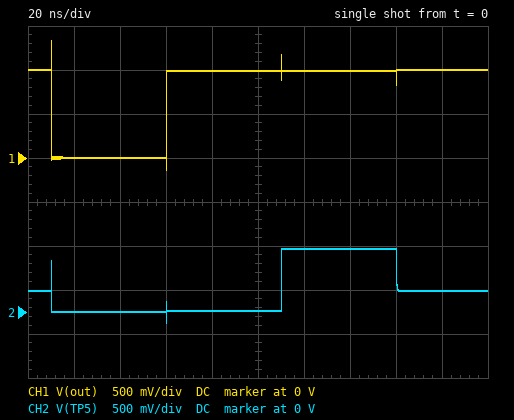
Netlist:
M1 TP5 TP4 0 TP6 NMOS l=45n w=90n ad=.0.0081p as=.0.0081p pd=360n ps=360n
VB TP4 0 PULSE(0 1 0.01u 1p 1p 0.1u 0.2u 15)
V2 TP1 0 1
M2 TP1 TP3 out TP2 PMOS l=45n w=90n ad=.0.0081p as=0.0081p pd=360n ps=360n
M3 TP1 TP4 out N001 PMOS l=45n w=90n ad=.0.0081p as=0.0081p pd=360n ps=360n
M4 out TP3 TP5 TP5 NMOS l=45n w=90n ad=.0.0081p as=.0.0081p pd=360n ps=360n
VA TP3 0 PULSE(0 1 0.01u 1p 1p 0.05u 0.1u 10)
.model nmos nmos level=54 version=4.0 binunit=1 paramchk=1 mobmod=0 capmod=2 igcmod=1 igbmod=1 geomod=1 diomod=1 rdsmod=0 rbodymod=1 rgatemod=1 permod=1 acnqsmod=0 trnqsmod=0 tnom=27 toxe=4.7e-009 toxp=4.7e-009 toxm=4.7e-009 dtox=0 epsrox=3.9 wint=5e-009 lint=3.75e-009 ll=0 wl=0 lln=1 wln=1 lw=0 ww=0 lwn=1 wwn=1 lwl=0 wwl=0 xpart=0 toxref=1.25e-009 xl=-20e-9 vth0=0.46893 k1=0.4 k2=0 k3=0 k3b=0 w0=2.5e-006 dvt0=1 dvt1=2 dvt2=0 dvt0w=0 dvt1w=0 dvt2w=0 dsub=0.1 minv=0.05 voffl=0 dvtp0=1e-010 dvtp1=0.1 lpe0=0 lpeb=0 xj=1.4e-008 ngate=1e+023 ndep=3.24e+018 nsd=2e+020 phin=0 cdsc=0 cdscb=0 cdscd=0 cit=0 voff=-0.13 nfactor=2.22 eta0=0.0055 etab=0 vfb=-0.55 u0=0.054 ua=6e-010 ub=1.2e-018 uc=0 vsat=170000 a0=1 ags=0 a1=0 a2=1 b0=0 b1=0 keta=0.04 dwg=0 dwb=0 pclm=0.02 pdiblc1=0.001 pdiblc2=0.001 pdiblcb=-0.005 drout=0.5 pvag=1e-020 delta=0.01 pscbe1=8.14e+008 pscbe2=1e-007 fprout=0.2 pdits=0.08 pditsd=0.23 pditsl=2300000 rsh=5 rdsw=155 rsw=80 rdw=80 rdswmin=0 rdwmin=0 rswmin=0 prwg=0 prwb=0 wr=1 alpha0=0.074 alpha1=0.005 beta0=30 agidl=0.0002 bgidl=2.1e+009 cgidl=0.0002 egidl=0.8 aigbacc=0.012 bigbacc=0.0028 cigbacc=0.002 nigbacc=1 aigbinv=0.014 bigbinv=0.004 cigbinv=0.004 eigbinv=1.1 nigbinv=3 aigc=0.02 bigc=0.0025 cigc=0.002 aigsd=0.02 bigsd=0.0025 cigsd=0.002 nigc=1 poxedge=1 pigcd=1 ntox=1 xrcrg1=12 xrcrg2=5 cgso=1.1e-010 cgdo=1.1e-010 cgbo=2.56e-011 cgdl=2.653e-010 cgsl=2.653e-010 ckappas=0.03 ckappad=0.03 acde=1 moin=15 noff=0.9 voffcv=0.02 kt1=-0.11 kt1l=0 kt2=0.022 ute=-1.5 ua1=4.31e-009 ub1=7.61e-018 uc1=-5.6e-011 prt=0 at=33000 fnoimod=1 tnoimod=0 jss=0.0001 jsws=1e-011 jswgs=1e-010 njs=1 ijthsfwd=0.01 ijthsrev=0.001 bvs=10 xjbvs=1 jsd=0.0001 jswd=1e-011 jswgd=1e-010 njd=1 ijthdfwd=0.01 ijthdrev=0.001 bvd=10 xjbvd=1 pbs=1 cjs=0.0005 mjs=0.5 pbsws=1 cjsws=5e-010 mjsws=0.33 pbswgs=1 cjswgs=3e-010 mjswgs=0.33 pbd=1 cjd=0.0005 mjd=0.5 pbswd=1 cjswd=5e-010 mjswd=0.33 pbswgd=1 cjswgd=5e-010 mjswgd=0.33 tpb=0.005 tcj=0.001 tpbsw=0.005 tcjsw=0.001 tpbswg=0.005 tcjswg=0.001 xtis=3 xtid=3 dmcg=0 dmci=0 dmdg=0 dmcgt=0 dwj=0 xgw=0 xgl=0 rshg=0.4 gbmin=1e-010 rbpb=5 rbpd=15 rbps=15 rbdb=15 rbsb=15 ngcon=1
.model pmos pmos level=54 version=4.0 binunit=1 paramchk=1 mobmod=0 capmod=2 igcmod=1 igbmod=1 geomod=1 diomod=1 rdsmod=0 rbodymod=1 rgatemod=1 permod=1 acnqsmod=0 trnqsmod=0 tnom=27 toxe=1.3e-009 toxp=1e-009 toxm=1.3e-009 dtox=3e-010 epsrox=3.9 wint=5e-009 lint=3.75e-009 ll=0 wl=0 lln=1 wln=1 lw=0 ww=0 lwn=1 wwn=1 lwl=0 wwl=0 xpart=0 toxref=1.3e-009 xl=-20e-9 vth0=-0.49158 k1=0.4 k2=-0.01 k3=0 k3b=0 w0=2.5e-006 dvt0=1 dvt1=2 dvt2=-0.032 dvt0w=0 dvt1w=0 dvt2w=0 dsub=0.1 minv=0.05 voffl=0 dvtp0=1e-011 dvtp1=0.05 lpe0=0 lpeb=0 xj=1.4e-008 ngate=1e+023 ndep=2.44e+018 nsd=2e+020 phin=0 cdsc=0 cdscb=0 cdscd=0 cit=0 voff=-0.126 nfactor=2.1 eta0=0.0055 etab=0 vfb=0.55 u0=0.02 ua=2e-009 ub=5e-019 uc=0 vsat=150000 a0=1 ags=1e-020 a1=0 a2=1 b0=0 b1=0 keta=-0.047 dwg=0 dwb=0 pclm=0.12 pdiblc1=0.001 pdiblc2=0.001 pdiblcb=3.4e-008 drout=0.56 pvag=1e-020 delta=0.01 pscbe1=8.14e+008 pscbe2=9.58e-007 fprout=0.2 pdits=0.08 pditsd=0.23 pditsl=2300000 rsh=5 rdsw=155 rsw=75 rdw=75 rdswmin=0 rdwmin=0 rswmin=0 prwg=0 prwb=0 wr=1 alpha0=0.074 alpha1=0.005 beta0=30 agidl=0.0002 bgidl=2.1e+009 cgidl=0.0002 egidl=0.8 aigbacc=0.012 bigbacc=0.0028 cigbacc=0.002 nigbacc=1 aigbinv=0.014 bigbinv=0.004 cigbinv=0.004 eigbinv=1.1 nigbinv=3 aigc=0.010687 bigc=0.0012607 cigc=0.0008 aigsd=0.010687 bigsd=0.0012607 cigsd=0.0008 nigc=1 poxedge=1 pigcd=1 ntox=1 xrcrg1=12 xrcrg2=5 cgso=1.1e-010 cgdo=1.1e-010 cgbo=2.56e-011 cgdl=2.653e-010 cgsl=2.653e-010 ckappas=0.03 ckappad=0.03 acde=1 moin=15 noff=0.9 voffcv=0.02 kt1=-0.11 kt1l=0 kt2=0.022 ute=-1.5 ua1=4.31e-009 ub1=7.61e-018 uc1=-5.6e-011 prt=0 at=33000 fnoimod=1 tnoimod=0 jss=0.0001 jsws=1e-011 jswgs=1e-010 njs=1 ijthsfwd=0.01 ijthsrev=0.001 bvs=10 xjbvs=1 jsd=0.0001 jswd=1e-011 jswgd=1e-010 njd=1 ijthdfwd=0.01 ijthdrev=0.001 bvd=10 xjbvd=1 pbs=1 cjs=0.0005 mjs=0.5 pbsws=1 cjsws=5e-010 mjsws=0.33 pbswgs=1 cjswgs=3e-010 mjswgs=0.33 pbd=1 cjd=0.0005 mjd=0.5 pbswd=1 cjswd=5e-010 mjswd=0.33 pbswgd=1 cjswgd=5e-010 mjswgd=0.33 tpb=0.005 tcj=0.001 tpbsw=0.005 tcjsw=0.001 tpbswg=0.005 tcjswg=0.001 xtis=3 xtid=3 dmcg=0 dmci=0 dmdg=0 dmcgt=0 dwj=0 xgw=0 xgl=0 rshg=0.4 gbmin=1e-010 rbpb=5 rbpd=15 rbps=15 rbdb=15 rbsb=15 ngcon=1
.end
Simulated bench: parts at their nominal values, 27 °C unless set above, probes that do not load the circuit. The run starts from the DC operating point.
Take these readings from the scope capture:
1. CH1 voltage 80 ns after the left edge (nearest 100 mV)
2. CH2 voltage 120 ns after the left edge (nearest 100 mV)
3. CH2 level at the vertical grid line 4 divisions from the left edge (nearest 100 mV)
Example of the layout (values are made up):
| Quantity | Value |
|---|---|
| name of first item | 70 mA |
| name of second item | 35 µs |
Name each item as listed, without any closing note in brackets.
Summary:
| Quantity | Value |
|---|---|
| CH1 voltage 80 ns after the left edge | 1.0 V |
| CH2 voltage 120 ns after the left edge | 700 mV |
| CH2 level at the vertical grid line 4 divisions from the left edge | 0 V |
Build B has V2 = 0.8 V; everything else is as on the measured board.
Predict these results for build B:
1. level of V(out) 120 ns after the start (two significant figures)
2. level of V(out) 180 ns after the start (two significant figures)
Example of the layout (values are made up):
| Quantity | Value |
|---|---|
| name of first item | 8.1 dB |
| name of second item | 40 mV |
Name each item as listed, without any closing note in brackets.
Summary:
| Quantity | Value |
|---|---|
| level of V(out) 120 ns after the start | 790 mV |
| level of V(out) 180 ns after the start | 800 mV |
